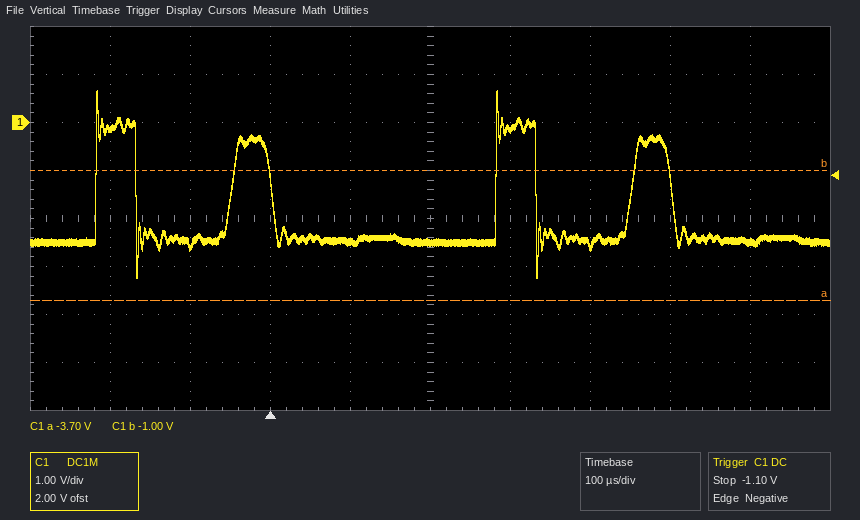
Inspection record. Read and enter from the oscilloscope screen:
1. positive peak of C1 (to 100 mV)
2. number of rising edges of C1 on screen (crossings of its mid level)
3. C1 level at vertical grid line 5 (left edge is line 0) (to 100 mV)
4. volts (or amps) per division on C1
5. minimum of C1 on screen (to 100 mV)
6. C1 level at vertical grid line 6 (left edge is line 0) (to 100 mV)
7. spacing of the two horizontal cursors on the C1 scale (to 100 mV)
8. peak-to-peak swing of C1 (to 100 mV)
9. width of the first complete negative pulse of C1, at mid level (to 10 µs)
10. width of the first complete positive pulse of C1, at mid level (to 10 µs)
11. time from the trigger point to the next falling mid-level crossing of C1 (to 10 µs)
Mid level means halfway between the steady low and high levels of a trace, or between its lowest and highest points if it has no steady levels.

700 mV
4
-2.5 V
1 V
-3.2 V
-100 mV
2.7 V
3.9 V
120 µs
50 µs
330 µs
